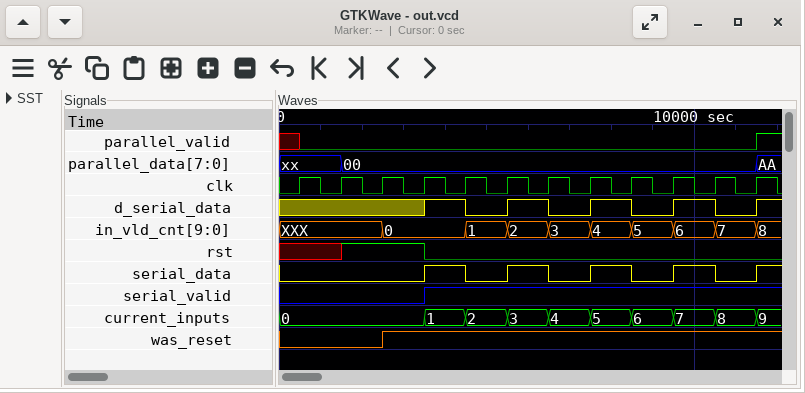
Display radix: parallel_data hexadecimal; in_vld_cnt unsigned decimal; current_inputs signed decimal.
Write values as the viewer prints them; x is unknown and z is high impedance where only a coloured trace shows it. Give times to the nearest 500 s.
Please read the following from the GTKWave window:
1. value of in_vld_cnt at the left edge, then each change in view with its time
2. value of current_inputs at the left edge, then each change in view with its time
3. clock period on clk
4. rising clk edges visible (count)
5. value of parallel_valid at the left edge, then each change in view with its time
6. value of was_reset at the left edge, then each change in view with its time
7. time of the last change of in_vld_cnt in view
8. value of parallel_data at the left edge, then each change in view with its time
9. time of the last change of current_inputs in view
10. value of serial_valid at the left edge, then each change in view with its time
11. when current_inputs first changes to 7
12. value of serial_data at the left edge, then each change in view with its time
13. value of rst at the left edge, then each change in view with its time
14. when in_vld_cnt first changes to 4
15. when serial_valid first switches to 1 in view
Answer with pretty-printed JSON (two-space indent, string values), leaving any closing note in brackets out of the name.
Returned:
{
  "value of in_vld_cnt at the left edge, then each change in view with its time": "XXX, 0 at 2500 s, 1 at 4500 s, 2 at 5500 s, 3 at 6500 s, 4 at 7500 s, 5 at 8500 s, 6 at 9500 s, 7 at 10500 s, 8 at 11500 s",
  "value of current_inputs at the left edge, then each change in view with its time": "0, 1 at 3500 s, 2 at 4500 s, 3 at 5500 s, 4 at 6500 s, 5 at 7500 s, 6 at 8500 s, 7 at 9500 s, 8 at 10500 s, 9 at 11500 s",
  "clock period on clk": "1000 s",
  "rising clk edges visible": "12",
  "value of parallel_valid at the left edge, then each change in view with its time": "x, 0 at 500 s, 1 at 11500 s",
  "value of was_reset at the left edge, then each change in view with its time": "0, 1 at 2500 s",
  "time of the last change of in_vld_cnt in view": "11500 s",
  "value of parallel_data at the left edge, then each change in view with its time": "xx, 00 at 1500 s, AA at 11500 s",
  "time of the last change of current_inputs in view": "11500 s",
  "value of serial_valid at the left edge, then each change in view with its time": "0, 1 at 3500 s",
  "when current_inputs first changes to 7": "9500 s",
  "value of serial_data at the left edge, then each change in view with its time": "0, 1 at 3500 s, 0 at 4500 s, 1 at 5500 s, 0 at 6500 s, 1 at 7500 s, 0 at 8500 s, 1 at 9500 s, 0 at 10500 s, 1 at 11500 s",
  "value of rst at the left edge, then each change in view with its time": "x, 1 at 1500 s, 0 at 3500 s",
  "when in_vld_cnt first changes to 4": "7500 s",
  "when serial_valid first switches to 1 in view": "3500 s"
}
